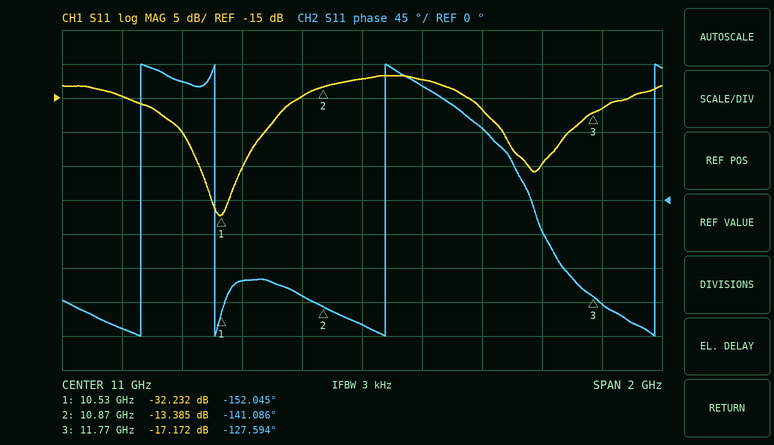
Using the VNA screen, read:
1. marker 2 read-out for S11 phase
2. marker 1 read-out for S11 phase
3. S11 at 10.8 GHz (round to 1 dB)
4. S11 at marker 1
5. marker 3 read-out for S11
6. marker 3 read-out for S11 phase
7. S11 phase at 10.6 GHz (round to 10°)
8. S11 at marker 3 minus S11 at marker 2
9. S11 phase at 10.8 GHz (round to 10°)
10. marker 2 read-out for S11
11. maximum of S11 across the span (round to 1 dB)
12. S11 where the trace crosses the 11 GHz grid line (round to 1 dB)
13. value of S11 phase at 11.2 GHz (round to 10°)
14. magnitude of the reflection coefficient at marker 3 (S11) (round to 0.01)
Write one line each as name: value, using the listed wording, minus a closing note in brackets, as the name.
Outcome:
marker 2 read-out for S11 phase: -141.086°
marker 1 read-out for S11 phase: -152.045°
S11 at 10.8 GHz: -15 dB
S11 at marker 1: -32.232 dB
marker 3 read-out for S11: -17.172 dB
marker 3 read-out for S11 phase: -127.594°
S11 phase at 10.6 GHz: -110°
S11 at marker 3 minus S11 at marker 2: -3.787 dB
S11 phase at 10.8 GHz: -130°
marker 2 read-out for S11: -13.385 dB
maximum of S11 across the span: -12 dB
S11 where the trace crosses the 11 GHz grid line: -12 dB
value of S11 phase at 11.2 GHz: 150°
magnitude of the reflection coefficient at marker 3 (S11): 0.14
